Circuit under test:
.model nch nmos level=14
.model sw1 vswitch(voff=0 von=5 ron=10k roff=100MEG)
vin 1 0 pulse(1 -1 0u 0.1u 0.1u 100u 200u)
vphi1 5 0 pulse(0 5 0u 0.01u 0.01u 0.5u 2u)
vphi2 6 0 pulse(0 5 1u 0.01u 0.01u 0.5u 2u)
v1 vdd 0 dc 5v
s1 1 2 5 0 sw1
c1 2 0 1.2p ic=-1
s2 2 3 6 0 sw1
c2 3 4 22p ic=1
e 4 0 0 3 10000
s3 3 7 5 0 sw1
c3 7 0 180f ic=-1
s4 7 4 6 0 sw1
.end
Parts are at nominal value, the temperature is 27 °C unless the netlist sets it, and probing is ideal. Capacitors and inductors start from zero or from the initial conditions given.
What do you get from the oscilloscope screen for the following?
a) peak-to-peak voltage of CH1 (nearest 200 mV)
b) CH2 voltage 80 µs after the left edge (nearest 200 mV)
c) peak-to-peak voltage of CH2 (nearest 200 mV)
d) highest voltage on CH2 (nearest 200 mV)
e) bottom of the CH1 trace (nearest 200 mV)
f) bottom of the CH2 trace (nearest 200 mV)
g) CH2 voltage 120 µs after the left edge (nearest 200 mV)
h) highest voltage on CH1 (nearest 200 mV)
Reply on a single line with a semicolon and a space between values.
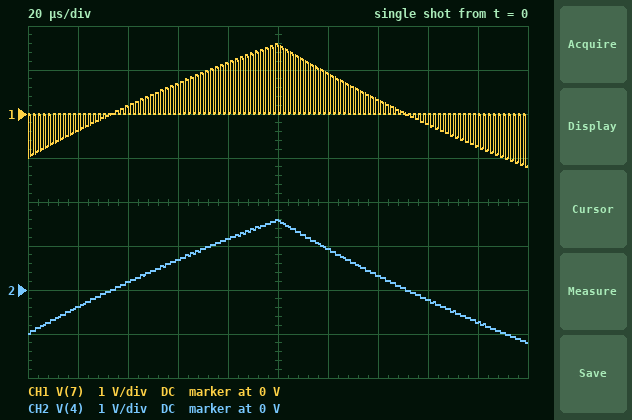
2.8 V; 1.2 V; 2.8 V; 1.6 V; -1.2 V; -1.2 V; 1.0 V; 1.6 V
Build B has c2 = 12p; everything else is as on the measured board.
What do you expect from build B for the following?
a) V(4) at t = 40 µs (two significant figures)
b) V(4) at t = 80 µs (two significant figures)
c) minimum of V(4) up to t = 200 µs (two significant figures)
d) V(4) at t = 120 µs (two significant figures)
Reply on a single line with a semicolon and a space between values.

1.0 V; 2.5 V; -2.1 V; 1.7 V
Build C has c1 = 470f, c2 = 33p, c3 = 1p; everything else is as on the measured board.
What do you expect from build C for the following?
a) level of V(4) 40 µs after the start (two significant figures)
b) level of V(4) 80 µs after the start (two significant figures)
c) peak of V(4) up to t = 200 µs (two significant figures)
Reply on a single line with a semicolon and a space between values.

-320 mV; 50 mV; 160 mV
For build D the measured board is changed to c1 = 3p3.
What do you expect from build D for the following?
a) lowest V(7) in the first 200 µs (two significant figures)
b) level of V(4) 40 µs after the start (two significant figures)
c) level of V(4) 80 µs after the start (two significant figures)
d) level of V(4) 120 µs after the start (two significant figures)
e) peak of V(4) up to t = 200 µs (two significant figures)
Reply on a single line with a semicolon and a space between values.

-2.6 V; 1.9 V; 4.4 V; 3.6 V; 5.5 V
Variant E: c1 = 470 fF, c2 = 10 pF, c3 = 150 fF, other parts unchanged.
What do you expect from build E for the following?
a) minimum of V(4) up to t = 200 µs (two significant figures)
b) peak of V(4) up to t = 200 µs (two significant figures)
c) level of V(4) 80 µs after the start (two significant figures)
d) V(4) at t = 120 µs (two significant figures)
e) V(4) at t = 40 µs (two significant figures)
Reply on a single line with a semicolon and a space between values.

-1.1 V; 1.2 V; 900 mV; 590 mV; 100 mV
